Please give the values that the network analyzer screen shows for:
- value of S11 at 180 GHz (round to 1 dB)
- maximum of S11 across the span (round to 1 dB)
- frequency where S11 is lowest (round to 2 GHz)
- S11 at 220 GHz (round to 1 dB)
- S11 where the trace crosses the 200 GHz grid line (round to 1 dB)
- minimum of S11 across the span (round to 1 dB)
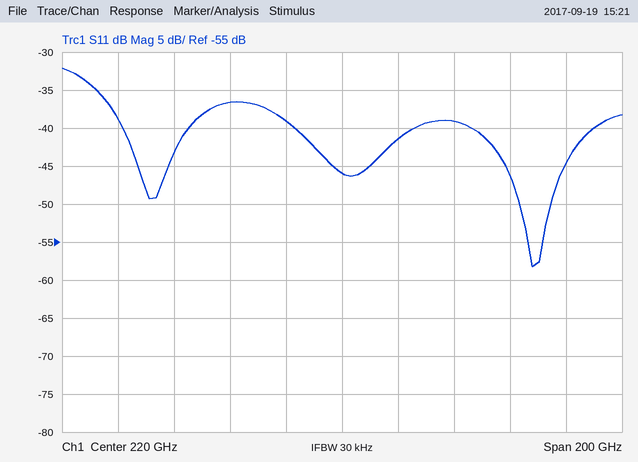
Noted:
-37 dB
-32 dB
288 GHz
-46 dB
-39 dB
-58 dB
